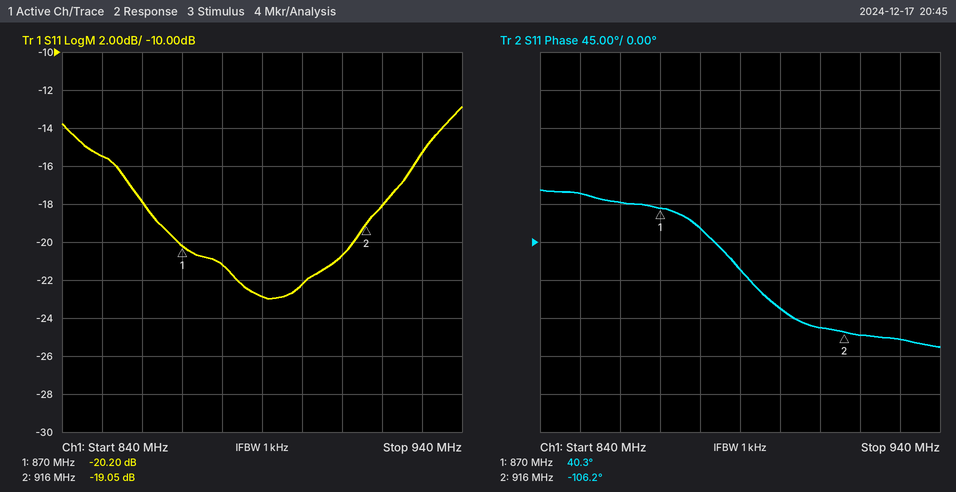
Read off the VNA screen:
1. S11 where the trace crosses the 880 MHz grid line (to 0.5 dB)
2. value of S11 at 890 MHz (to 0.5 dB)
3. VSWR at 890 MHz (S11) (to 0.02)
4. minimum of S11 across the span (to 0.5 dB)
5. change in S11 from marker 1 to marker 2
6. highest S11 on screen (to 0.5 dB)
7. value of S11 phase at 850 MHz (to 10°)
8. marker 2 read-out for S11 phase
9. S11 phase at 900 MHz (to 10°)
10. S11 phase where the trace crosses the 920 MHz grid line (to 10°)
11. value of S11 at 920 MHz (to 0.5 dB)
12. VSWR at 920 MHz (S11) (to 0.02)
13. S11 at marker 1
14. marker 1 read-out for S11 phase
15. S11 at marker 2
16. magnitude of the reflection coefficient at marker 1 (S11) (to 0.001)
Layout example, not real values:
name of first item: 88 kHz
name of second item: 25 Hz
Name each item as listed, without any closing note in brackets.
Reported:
S11 where the trace crosses the 880 MHz grid line: -21.0 dB
value of S11 at 890 MHz: -23.0 dB
VSWR at 890 MHz (S11): 1.16
minimum of S11 across the span: -23.0 dB
change in S11 from marker 1 to marker 2: 1.15 dB
highest S11 on screen: -13.0 dB
value of S11 phase at 850 MHz: 60°
marker 2 read-out for S11 phase: -106.2°
S11 phase at 900 MHz: -80°
S11 phase where the trace crosses the 920 MHz grid line: -110°
value of S11 at 920 MHz: -18.0 dB
VSWR at 920 MHz (S11): 1.28
S11 at marker 1: -20.20 dB
marker 1 read-out for S11 phase: 40.3°
S11 at marker 2: -19.05 dB
magnitude of the reflection coefficient at marker 1 (S11): 0.098
